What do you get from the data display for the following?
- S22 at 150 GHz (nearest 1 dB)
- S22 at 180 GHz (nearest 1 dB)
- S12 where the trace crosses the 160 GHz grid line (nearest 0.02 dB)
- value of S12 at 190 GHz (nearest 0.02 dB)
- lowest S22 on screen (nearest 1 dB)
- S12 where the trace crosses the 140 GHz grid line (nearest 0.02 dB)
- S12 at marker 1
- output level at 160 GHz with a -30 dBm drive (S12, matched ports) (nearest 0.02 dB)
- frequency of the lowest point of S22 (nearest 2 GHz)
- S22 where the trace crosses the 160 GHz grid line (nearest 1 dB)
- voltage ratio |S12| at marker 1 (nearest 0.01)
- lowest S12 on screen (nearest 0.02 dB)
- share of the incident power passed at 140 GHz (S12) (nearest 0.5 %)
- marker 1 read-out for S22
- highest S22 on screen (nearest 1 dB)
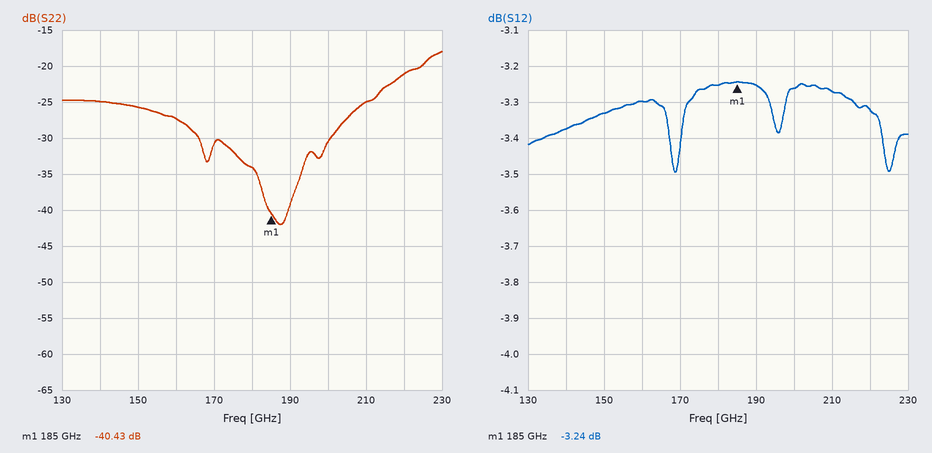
-26 dB
-34 dB
-3.30 dB
-3.26 dB
-42 dB
-3.38 dB
-3.24 dB
-33.30 dBm
188 GHz
-27 dB
0.69
-3.50 dB
46.0 %
-40.43 dB
-18 dB
